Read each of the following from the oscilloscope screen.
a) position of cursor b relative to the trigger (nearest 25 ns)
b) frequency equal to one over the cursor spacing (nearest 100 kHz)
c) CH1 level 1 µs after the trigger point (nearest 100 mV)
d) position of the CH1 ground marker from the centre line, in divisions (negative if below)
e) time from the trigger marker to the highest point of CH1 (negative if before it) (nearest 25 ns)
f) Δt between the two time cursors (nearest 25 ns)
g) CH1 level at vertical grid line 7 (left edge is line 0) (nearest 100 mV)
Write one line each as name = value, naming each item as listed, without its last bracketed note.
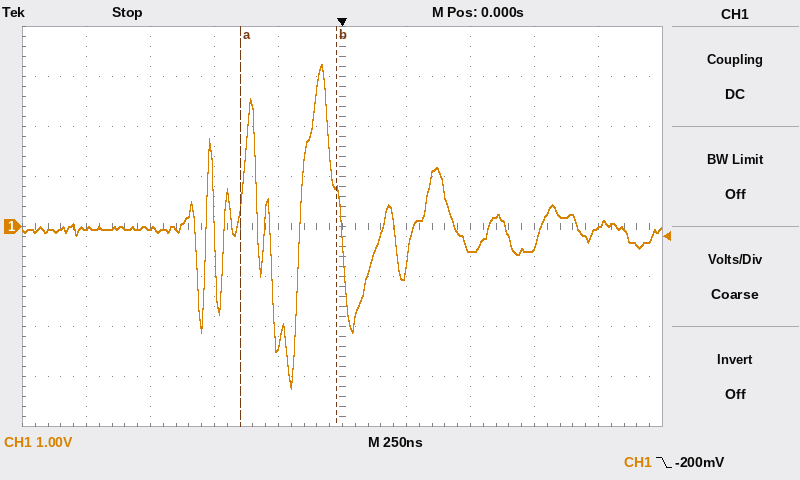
position of cursor b relative to the trigger = -25 ns
frequency equal to one over the cursor spacing = 2.7 MHz
CH1 level 1 µs after the trigger point = 0.0 V
position of the CH1 ground marker from the centre line, in divisions = 0.0 div
time from the trigger marker to the highest point of CH1 (negative if before it) = -75 ns
Δt between the two time cursors = 375 ns
CH1 level at vertical grid line 7 (left edge is line 0) = -500 mV
